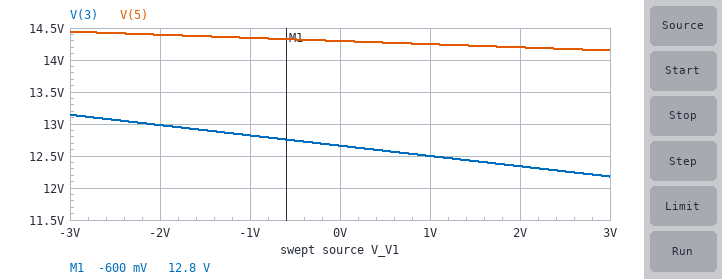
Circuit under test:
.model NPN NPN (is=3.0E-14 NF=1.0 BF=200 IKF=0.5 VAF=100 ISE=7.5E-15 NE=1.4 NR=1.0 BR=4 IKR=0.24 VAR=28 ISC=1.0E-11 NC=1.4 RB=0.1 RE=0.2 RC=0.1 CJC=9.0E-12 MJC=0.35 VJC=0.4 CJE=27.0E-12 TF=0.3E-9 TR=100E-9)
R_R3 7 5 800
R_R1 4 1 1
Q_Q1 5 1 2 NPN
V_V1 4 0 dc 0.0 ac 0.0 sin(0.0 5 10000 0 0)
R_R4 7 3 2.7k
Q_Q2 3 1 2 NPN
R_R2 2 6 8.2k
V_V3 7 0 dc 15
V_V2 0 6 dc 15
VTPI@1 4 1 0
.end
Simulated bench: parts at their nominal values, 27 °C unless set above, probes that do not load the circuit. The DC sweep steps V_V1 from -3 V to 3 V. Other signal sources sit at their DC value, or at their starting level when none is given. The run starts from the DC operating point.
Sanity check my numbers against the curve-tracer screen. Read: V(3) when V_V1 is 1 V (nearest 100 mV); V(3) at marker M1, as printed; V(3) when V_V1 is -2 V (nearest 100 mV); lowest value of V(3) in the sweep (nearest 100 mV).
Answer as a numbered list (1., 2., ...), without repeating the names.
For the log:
1. 12.5 V
2. 12.8 V
3. 13.0 V
4. 12.2 V
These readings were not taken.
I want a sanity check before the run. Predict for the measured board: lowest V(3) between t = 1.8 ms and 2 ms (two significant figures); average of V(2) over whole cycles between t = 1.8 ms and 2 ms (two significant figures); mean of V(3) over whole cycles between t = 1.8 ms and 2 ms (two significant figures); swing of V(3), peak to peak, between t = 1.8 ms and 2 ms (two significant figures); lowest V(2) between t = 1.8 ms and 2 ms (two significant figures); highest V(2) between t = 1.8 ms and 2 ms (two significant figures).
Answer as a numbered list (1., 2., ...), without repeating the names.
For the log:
1. 12 V
2. -620 mV
3. 13 V
4. 1.6 V
5. -5.6 V
6. 4.4 V
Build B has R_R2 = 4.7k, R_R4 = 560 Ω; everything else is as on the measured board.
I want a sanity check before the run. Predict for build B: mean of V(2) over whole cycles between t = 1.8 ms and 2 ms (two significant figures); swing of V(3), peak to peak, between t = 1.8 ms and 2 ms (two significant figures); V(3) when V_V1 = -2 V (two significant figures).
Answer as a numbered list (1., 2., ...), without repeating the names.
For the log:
1. -630 mV
2. 590 mV
3. 14 V
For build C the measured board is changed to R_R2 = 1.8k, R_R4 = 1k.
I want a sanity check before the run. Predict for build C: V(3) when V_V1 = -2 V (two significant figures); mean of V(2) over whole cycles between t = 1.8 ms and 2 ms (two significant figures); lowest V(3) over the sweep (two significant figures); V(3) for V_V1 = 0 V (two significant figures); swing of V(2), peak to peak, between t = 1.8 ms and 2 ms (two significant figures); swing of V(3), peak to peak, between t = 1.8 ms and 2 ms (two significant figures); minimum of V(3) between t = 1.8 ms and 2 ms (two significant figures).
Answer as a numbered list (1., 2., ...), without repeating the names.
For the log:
1. 12 V
2. -660 mV
3. 10 V
4. 11 V
5. 10 V
6. 2.7 V
7. 9.7 V
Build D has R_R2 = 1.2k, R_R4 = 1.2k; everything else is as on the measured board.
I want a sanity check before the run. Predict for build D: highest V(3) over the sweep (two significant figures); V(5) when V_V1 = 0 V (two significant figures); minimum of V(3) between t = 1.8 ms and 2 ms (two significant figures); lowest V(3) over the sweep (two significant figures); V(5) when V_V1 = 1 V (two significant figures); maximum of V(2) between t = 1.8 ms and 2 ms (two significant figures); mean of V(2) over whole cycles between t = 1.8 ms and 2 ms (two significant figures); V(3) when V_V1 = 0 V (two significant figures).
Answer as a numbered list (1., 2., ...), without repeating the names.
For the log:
1. 9.4 V
2. 10 V
3. 5.5 V
4. 6.5 V
5. 9.9 V
6. 4.3 V
7. -670 mV
8. 7.9 V
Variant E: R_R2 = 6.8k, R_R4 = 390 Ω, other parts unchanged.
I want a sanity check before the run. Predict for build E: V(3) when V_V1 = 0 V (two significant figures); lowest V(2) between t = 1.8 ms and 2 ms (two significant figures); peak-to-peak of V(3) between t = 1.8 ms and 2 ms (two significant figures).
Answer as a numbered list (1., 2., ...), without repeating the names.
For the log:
1. 15 V
2. -5.6 V
3. 290 mV
